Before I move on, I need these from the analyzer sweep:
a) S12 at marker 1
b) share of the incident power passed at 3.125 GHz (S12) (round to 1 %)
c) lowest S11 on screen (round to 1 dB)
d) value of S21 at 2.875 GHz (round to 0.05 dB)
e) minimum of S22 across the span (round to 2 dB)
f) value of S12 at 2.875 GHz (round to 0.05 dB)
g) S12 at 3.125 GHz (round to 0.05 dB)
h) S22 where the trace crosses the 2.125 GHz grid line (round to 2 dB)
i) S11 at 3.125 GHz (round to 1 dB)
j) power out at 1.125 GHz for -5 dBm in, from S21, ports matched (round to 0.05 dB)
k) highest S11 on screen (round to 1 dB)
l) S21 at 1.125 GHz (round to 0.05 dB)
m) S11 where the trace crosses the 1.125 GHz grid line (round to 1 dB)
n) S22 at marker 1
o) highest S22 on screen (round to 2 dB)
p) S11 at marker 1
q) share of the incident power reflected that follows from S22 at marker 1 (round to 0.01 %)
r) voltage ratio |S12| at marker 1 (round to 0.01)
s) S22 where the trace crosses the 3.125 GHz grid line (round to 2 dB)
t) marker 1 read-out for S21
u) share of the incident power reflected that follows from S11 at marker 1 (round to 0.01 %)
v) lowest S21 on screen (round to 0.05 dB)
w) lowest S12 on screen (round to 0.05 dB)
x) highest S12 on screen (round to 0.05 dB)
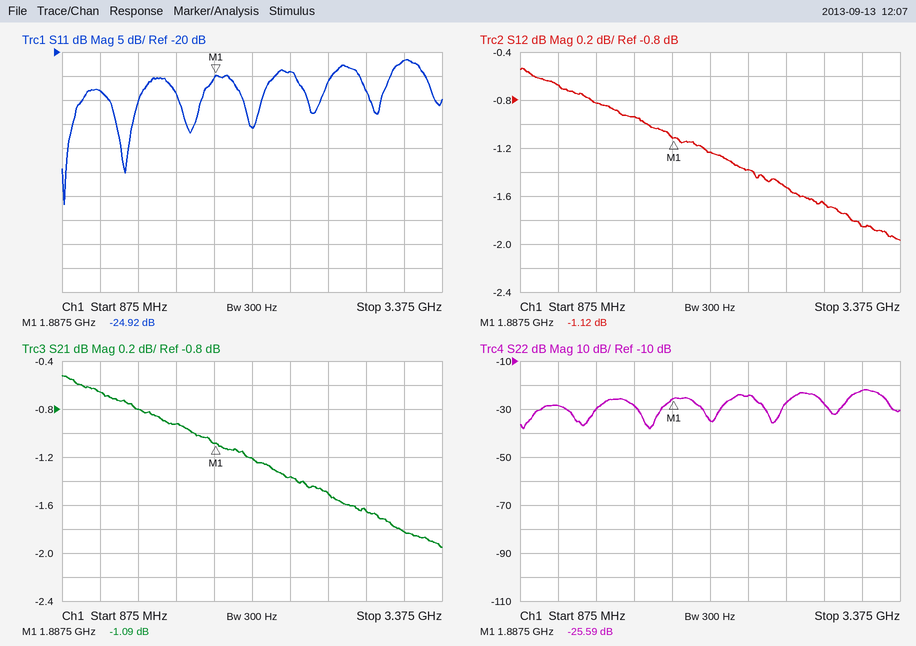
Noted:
-1.12 dB
65 %
-52 dB
-1.65 dB
-38 dB
-1.65 dB
-1.85 dB
-34 dB
-22 dB
-5.65 dBm
-22 dB
-0.65 dB
-28 dB
-25.59 dB
-22 dB
-24.92 dB
0.28 %
0.88
-22 dB
-1.09 dB
0.32 %
-1.95 dB
-1.95 dB
-0.55 dB
